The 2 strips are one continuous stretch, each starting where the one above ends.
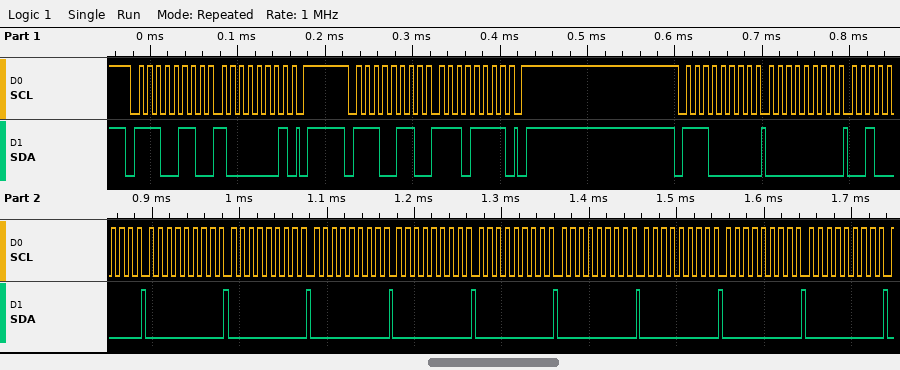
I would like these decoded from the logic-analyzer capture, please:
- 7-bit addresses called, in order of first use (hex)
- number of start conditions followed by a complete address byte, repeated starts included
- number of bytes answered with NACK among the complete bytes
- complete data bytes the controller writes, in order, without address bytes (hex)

0x73 0x70
3
0
81 EF 00 20 00 00 00 00 00 00 00 00 00
